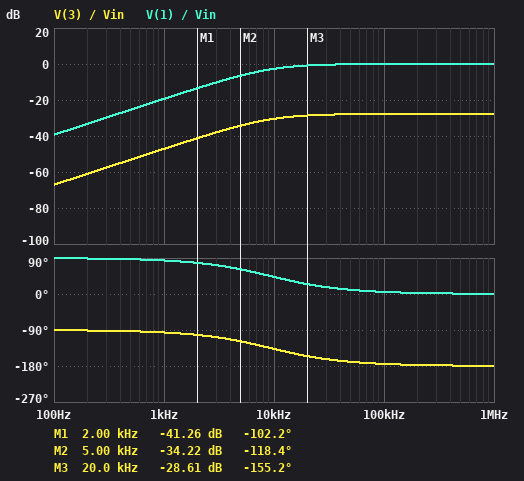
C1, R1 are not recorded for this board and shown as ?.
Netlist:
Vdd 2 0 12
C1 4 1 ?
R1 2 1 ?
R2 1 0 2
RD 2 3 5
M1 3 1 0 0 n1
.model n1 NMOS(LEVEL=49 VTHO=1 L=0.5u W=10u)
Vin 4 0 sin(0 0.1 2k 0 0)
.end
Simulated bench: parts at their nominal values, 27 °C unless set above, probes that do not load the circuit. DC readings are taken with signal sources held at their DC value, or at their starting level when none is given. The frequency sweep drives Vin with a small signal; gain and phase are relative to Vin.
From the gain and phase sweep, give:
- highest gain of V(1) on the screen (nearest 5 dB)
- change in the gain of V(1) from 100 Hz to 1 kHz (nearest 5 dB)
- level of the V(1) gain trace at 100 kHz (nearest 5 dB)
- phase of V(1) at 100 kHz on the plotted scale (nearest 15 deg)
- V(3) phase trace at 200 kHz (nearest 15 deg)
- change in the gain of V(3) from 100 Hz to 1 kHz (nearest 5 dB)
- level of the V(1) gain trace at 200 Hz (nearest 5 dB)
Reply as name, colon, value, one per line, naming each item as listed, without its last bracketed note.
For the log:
highest gain of V(1) on the screen: 0 dB
change in the gain of V(1) from 100 Hz to 1 kHz: 20 dB
level of the V(1) gain trace at 100 kHz: 0 dB
phase of V(1) at 100 kHz on the plotted scale: 0 deg
V(3) phase trace at 200 kHz: -180 deg
change in the gain of V(3) from 100 Hz to 1 kHz: 20 dB
level of the V(1) gain trace at 200 Hz: -35 dB
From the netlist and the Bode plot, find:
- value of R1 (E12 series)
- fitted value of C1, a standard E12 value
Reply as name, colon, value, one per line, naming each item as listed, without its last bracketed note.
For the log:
value of R1: 2.7 Ω
fitted value of C1, a standard E12 value: 15 µF
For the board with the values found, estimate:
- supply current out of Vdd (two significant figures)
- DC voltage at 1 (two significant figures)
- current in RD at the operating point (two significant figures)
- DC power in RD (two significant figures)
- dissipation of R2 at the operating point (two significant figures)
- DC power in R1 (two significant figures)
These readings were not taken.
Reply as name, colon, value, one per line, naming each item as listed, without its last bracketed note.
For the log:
supply current out of Vdd: 2.6 A
DC voltage at 1: 5.1 V
current in RD at the operating point: 40 mA
DC power in RD: 8.2 mW
dissipation of R2 at the operating point: 13 W
DC power in R1: 18 W
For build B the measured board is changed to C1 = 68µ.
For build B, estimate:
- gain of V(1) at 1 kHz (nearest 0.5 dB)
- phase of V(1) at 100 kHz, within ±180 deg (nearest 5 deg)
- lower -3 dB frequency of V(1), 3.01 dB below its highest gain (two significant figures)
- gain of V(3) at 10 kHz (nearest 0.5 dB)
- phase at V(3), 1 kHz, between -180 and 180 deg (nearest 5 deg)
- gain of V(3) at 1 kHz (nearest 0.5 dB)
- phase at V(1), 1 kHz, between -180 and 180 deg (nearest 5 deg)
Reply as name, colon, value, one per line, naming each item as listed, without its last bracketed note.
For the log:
gain of V(1) at 1 kHz: -7.0 dB
phase of V(1) at 100 kHz, within ±180 deg: 0 deg
lower -3 dB frequency of V(1), 3.01 dB below its highest gain: 2.0 kHz
gain of V(3) at 10 kHz: -28.0 dB
phase at V(3), 1 kHz, between -180 and 180 deg: -115 deg
gain of V(3) at 1 kHz: -35.0 dB
phase at V(1), 1 kHz, between -180 and 180 deg: 65 deg
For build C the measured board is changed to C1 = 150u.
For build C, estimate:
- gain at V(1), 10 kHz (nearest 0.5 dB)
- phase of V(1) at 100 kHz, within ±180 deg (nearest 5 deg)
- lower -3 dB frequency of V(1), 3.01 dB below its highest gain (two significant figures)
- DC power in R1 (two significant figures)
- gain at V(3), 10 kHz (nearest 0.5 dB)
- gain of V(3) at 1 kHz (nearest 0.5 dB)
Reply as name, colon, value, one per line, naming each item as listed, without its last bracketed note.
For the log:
gain at V(1), 10 kHz: 0 dB
phase of V(1) at 100 kHz, within ±180 deg: 0 deg
lower -3 dB frequency of V(1), 3.01 dB below its highest gain: 920 Hz
DC power in R1: 18 W
gain at V(3), 10 kHz: -28.0 dB
gain of V(3) at 1 kHz: -30.5 dB
